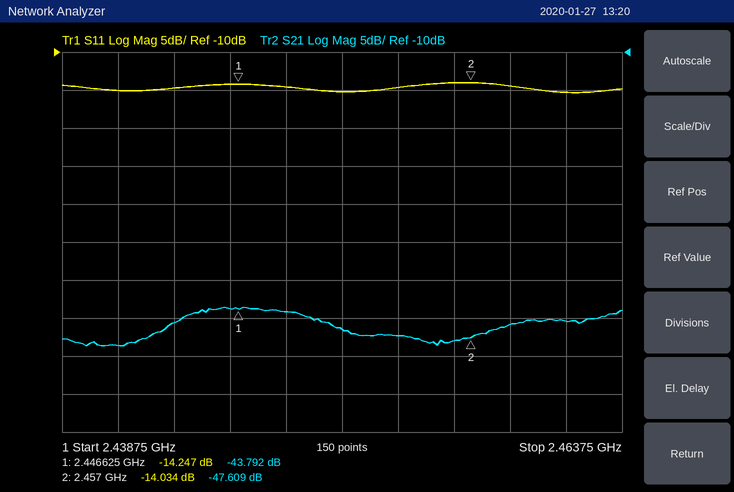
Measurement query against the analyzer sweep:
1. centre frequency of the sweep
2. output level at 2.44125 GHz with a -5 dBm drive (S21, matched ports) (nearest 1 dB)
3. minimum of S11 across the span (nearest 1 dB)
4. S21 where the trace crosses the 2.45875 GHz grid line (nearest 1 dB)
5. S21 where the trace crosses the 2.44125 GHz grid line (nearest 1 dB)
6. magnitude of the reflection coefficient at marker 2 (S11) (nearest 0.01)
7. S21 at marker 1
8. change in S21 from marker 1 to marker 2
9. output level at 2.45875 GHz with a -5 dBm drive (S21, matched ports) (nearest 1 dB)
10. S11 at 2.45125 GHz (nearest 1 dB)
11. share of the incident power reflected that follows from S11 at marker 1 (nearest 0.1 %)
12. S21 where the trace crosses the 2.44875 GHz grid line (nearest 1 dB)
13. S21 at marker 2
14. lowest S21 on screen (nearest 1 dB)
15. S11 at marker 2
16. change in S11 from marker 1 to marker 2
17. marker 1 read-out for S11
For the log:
2.45125 GHz
-54 dBm
-15 dB
-46 dB
-49 dB
0.20
-43.792 dB
-3.817 dB
-51 dBm
-15 dB
3.8 %
-44 dB
-47.609 dB
-49 dB
-14.034 dB
0.213 dB
-14.247 dB
